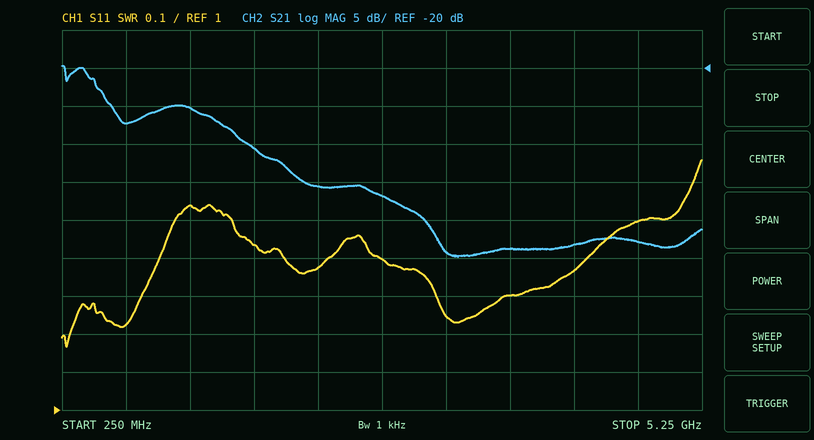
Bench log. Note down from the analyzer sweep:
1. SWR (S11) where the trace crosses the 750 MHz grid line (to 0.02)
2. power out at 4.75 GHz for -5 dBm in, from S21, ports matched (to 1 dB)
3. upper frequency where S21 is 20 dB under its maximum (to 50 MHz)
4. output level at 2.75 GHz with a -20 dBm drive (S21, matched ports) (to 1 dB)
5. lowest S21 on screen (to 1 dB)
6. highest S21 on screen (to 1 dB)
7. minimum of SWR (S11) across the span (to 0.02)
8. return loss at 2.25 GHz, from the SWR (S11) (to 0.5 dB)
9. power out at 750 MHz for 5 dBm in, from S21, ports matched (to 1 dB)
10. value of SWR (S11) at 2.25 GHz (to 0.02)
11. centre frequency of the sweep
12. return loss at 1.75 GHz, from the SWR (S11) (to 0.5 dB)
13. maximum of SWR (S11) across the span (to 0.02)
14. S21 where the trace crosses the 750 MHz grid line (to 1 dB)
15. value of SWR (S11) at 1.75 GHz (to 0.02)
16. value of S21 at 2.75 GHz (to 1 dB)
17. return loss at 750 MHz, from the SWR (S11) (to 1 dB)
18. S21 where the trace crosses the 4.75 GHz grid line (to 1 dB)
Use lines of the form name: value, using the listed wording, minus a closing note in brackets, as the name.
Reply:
SWR (S11) where the trace crosses the 750 MHz grid line: 1.22
power out at 4.75 GHz for -5 dBm in, from S21, ports matched: -48 dBm
upper frequency where S21 is 20 dB under its maximum: 3.05 GHz
output level at 2.75 GHz with a -20 dBm drive (S21, matched ports): -57 dBm
lowest S21 on screen: -45 dB
highest S21 on screen: -20 dB
minimum of SWR (S11) across the span: 1.16
return loss at 2.25 GHz, from the SWR (S11): 16.0 dB
power out at 750 MHz for 5 dBm in, from S21, ports matched: -22 dBm
value of SWR (S11) at 2.25 GHz: 1.38
centre frequency of the sweep: 2.75 GHz
return loss at 1.75 GHz, from the SWR (S11): 15.0 dB
maximum of SWR (S11) across the span: 1.66
S21 where the trace crosses the 750 MHz grid line: -27 dB
value of SWR (S11) at 1.75 GHz: 1.44
value of S21 at 2.75 GHz: -37 dB
return loss at 750 MHz, from the SWR (S11): 20 dB
S21 where the trace crosses the 4.75 GHz grid line: -43 dB
